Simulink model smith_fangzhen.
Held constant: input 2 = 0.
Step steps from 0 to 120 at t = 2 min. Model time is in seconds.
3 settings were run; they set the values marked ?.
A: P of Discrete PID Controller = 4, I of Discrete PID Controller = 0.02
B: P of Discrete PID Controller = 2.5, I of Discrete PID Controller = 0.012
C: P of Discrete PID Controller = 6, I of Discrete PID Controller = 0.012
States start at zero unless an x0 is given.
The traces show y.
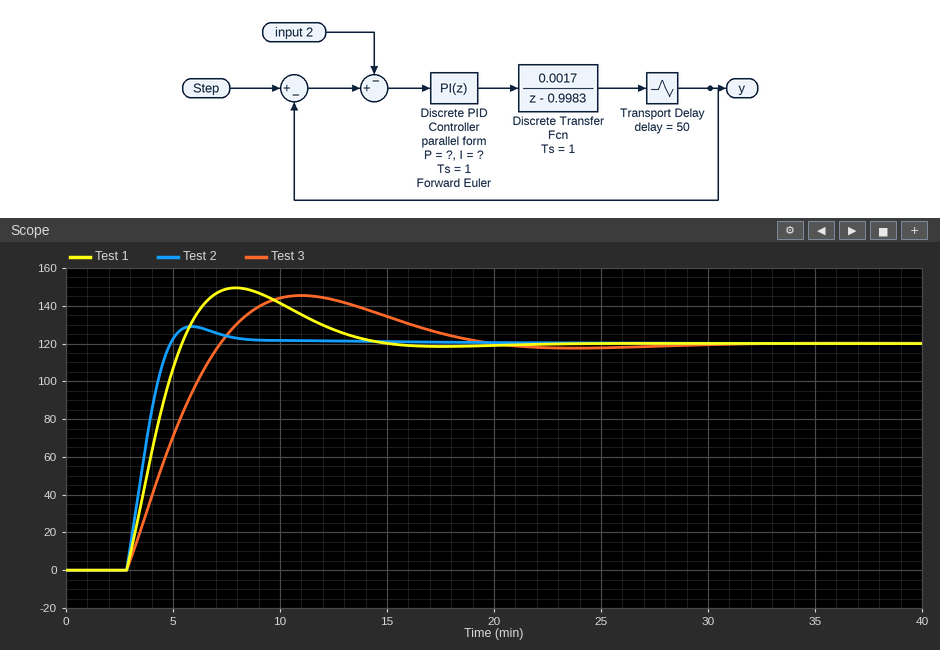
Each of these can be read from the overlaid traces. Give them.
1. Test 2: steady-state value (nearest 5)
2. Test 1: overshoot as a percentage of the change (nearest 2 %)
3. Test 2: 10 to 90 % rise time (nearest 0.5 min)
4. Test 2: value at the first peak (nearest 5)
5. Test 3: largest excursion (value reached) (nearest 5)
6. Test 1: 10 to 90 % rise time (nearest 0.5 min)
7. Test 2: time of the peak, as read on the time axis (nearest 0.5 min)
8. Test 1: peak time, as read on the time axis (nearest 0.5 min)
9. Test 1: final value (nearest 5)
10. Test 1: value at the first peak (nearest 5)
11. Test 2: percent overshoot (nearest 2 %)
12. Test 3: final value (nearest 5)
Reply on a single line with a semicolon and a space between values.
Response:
120; 24 %; 1.5 min; 130; 145; 2.0 min; 6.0 min; 8.0 min; 120; 150; 8 %; 120
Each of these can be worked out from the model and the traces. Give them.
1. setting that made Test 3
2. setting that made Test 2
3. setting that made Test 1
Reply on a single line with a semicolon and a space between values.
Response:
B; C; A
